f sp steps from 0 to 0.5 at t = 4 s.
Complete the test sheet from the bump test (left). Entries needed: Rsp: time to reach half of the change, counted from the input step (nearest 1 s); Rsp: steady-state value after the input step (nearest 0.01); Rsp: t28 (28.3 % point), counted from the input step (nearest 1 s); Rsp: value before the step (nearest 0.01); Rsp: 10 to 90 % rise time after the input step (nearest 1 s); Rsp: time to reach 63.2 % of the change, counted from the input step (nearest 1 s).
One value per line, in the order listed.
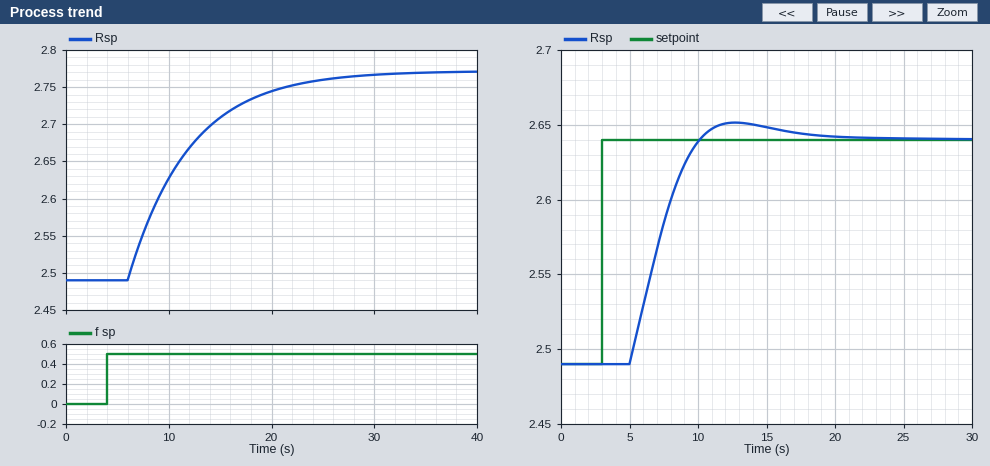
6 s
2.77
4 s
2.49
13 s
8 s
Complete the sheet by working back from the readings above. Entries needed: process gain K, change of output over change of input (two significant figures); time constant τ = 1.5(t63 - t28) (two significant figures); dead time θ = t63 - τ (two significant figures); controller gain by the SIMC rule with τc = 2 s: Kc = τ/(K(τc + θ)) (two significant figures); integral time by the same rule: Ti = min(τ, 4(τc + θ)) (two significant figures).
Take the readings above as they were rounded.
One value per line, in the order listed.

0.56
6.0 s
2.0 s
2.7
6.0 s
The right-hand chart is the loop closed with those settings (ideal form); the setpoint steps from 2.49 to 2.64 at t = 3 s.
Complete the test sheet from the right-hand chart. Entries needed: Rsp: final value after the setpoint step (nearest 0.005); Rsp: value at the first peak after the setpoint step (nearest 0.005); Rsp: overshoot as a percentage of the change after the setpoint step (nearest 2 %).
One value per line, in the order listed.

2.640
2.650
8 %
